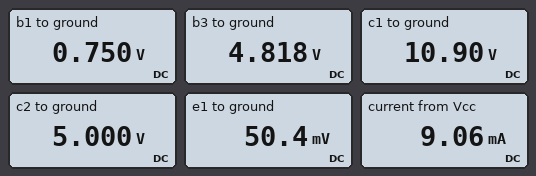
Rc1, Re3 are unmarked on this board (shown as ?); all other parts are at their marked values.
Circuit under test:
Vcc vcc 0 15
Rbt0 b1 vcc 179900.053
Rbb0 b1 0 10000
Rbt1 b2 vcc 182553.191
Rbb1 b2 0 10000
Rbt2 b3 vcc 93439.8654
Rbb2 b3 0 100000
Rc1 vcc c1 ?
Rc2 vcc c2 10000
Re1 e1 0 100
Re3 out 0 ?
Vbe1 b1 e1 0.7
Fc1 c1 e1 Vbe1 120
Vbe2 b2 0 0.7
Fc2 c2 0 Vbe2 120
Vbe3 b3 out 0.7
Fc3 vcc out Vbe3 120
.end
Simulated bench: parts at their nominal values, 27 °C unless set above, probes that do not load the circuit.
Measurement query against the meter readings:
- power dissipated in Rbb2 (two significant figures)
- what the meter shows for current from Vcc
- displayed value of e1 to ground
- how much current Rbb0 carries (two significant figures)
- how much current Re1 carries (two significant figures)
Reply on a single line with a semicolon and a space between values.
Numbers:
230 µW; 9.06 mA; 50.4 mV; 75 µA; 500 µA
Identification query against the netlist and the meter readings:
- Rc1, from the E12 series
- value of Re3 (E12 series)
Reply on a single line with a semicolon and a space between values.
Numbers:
8.2 kΩ; 560 Ω
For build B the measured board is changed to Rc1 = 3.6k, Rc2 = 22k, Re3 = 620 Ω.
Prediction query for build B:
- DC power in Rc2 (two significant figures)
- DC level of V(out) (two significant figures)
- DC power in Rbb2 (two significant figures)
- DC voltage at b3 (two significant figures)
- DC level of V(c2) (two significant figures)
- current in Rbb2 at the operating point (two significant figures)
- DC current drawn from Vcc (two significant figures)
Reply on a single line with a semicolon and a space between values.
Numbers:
22 mW; 4.3 V; 250 µW; 5.0 V; -7.0 V; 50 µA; 8.6 mA
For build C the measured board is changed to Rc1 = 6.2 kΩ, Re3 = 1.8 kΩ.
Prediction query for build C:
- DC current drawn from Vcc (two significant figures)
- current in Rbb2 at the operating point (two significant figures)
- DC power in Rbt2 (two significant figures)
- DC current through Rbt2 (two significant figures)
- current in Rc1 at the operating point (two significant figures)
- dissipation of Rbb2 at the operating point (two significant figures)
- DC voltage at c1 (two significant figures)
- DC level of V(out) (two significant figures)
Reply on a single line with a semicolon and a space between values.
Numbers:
4.9 mA; 65 µA; 780 µW; 91 µA; 500 µA; 420 µW; 12 V; 5.8 V
